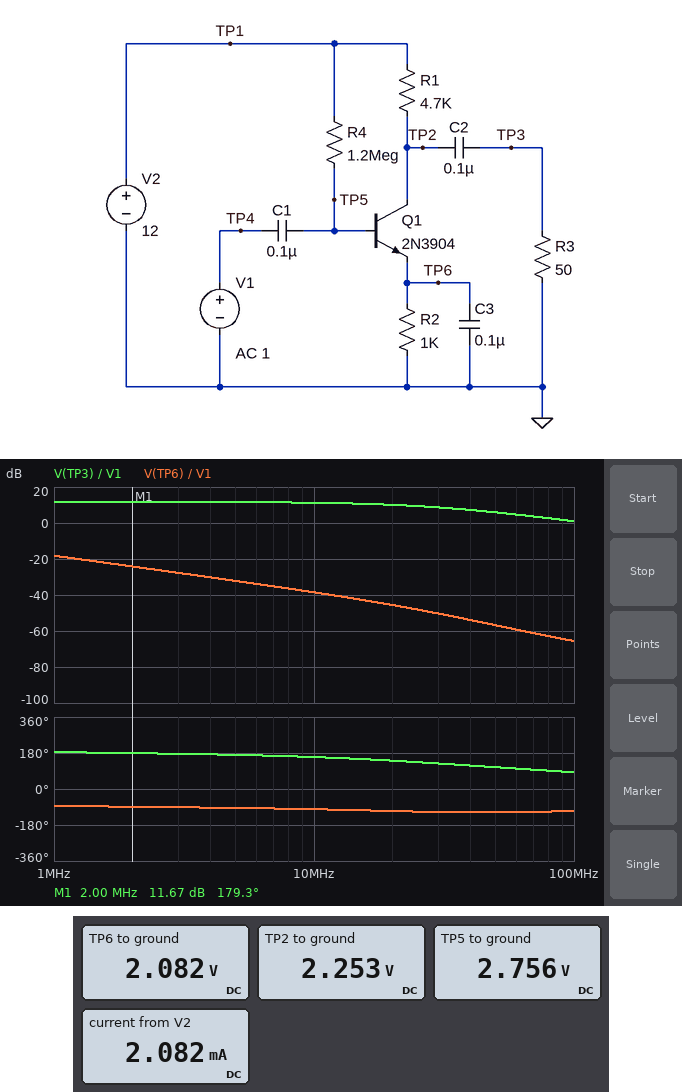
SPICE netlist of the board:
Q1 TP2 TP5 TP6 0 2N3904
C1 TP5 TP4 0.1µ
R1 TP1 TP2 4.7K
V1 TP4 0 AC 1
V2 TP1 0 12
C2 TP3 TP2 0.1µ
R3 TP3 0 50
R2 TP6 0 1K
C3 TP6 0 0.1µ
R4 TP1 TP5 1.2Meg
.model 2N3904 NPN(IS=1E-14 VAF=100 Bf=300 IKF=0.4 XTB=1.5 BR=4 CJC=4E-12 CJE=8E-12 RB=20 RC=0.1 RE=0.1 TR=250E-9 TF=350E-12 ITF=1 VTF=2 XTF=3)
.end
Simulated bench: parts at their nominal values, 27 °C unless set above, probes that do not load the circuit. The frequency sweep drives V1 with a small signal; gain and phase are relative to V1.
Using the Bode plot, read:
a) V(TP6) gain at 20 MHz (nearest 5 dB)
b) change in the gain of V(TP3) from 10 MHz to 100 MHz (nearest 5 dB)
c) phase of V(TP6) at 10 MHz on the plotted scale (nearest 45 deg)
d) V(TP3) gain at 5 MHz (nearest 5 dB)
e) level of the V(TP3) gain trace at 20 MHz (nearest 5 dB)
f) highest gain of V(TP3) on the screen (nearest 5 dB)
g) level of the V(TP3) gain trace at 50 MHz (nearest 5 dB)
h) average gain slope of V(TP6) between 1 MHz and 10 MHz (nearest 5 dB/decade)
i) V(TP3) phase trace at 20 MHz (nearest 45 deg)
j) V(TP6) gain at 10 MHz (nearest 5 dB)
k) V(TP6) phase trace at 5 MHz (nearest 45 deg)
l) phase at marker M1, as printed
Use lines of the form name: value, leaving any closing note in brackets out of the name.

V(TP6) gain at 20 MHz: -45 dB
change in the gain of V(TP3) from 10 MHz to 100 MHz: -10 dB
phase of V(TP6) at 10 MHz on the plotted scale: -90 deg
V(TP3) gain at 5 MHz: 10 dB
level of the V(TP3) gain trace at 20 MHz: 10 dB
highest gain of V(TP3) on the screen: 10 dB
level of the V(TP3) gain trace at 50 MHz: 5 dB
average gain slope of V(TP6) between 1 MHz and 10 MHz: -20 dB/decade
V(TP3) phase trace at 20 MHz: 135 deg
V(TP6) gain at 10 MHz: -40 dB
V(TP6) phase trace at 5 MHz: -90 deg
phase at marker M1, as printed: 179.3 deg
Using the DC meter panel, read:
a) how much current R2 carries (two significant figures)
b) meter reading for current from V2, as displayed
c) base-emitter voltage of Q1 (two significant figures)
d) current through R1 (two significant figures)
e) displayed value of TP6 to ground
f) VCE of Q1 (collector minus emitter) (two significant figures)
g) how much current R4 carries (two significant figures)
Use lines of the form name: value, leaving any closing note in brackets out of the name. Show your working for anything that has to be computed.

how much current R2 carries: (2.082 V) / 1 kΩ = 2.1 mA
meter reading for current from V2, as displayed: 2.082 mA
base-emitter voltage of Q1: 2.756 V - 2.082 V = 670 mV
current through R1: (12 V - 2.253 V) / 4.7 kΩ = 2.1 mA
displayed value of TP6 to ground: 2.082 V
VCE of Q1 (collector minus emitter): 2.253 V - 2.082 V = 170 mV
how much current R4 carries: (12 V - 2.756 V) / 1.2 MΩ = 7.7 µA
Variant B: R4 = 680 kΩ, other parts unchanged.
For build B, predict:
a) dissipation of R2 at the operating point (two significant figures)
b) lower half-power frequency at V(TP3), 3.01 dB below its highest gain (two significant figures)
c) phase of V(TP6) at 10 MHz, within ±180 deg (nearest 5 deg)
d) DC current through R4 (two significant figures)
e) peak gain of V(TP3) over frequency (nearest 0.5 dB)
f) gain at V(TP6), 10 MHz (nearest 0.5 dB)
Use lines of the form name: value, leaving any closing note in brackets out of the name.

dissipation of R2 at the operating point: 4.4 mW
lower half-power frequency at V(TP3), 3.01 dB below its highest gain: 120 kHz
phase of V(TP6) at 10 MHz, within ±180 deg: -115 deg
DC current through R4: 14 µA
peak gain of V(TP3) over frequency: 11.0 dB
gain at V(TP6), 10 MHz: -44.0 dB
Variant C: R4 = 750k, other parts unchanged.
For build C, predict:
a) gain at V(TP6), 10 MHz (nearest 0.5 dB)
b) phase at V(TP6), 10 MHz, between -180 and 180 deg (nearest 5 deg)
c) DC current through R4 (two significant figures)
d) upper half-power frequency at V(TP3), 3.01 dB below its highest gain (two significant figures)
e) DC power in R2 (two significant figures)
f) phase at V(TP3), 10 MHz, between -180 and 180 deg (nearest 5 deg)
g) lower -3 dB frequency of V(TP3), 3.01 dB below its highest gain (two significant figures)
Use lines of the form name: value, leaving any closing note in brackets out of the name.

gain at V(TP6), 10 MHz: -43.5 dB
phase at V(TP6), 10 MHz, between -180 and 180 deg: -115 deg
DC current through R4: 12 µA
upper half-power frequency at V(TP3), 3.01 dB below its highest gain: 5.7 MHz
DC power in R2: 4.4 mW
phase at V(TP3), 10 MHz, between -180 and 180 deg: 110 deg
lower -3 dB frequency of V(TP3), 3.01 dB below its highest gain: 120 kHz
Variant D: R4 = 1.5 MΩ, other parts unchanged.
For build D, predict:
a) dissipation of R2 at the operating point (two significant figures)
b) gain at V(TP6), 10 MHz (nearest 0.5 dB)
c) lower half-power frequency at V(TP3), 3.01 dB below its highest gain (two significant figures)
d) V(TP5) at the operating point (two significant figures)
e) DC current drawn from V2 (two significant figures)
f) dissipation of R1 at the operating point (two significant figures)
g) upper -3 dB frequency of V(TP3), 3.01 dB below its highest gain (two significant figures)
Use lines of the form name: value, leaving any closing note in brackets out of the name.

dissipation of R2 at the operating point: 3.6 mW
gain at V(TP6), 10 MHz: -39.0 dB
lower half-power frequency at V(TP3), 3.01 dB below its highest gain: 120 kHz
V(TP5) at the operating point: 2.6 V
DC current drawn from V2: 1.9 mA
dissipation of R1 at the operating point: 17 mW
upper -3 dB frequency of V(TP3), 3.01 dB below its highest gain: 140 MHz
